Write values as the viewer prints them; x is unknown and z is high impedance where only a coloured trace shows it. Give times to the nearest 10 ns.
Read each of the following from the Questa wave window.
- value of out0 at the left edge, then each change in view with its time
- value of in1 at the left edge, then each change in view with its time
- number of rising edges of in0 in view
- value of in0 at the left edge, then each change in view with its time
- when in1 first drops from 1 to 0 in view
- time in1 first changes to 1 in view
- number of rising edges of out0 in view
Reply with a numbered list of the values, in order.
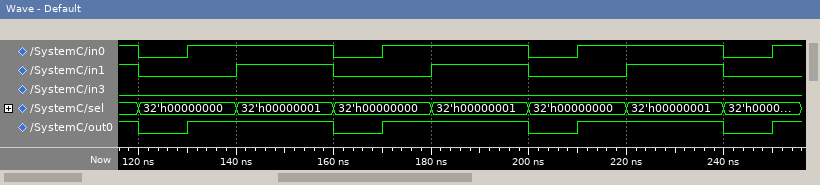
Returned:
1. 1, 0 at 120 ns, 1 at 130 ns, 0 at 160 ns, 1 at 170 ns, 0 at 200 ns, 1 at 210 ns, 0 at 240 ns, 1 at 250 ns
2. 1, 0 at 120 ns, 1 at 140 ns, 0 at 160 ns, 1 at 180 ns, 0 at 200 ns, 1 at 220 ns, 0 at 240 ns
3. 4
4. 1, 0 at 120 ns, 1 at 130 ns, 0 at 160 ns, 1 at 170 ns, 0 at 200 ns, 1 at 210 ns, 0 at 240 ns, 1 at 250 ns
5. 120 ns
6. 140 ns
7. 4
